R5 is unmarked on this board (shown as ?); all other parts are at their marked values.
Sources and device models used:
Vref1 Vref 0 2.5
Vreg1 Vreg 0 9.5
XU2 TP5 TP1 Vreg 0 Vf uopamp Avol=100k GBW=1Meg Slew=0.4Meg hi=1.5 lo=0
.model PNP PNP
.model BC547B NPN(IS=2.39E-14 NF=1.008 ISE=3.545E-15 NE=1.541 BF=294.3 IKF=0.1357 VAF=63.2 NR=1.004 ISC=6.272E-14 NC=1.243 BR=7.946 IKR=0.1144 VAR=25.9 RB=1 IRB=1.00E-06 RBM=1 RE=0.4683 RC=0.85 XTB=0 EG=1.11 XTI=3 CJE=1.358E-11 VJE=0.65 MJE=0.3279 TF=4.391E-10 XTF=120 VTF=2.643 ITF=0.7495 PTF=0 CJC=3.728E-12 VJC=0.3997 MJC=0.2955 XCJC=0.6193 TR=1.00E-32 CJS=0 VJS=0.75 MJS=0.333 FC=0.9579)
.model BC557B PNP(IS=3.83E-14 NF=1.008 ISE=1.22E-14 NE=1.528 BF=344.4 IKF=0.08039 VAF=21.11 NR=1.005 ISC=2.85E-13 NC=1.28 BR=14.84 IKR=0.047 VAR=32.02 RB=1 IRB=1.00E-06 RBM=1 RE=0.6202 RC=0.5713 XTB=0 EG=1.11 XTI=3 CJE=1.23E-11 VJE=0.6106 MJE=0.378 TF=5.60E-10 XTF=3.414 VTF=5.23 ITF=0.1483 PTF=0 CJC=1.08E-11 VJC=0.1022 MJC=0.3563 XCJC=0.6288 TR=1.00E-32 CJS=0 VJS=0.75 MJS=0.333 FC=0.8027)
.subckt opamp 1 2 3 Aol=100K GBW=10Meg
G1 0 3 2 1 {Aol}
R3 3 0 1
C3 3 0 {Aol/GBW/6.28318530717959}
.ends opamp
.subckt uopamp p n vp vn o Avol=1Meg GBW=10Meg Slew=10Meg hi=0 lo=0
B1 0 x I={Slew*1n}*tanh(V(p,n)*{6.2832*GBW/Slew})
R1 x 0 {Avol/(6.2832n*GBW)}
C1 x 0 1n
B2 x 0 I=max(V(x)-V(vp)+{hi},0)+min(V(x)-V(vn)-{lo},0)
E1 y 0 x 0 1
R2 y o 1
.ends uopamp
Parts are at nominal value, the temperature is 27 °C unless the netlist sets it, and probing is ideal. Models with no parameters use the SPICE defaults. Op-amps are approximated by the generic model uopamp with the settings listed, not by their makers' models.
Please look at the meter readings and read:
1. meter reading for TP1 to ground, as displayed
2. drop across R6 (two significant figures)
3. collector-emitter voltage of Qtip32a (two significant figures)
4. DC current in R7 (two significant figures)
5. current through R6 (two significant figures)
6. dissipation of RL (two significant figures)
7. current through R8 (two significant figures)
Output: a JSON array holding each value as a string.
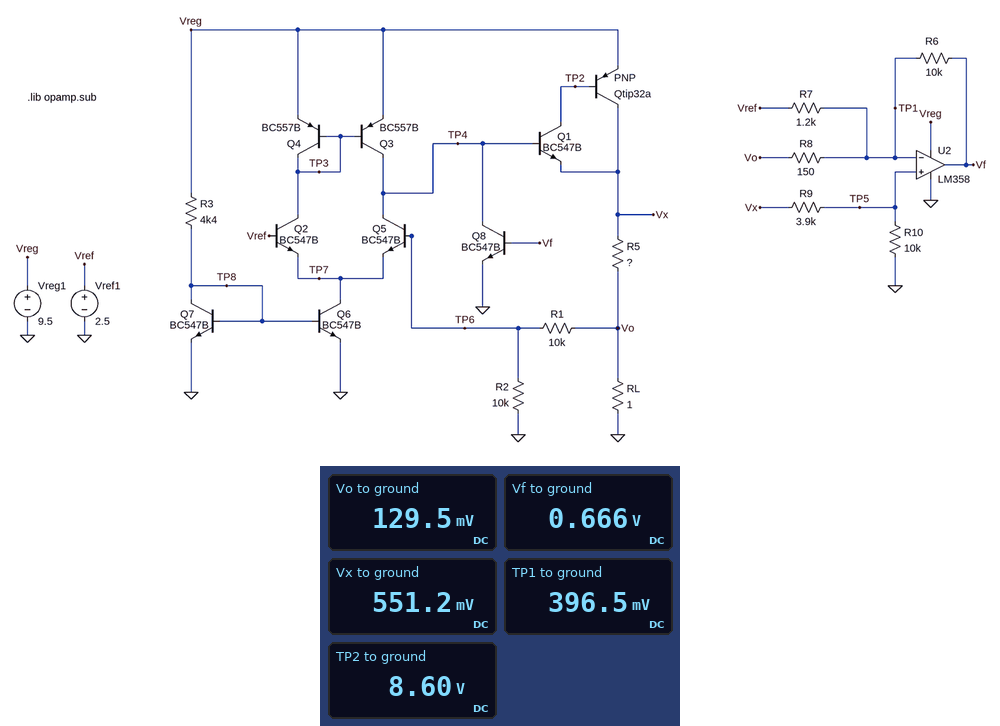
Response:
["396.5 mV", "270 mV", "-8.9 V", "1.8 mA", "27 µA", "17 mW", "1.8 mA"]
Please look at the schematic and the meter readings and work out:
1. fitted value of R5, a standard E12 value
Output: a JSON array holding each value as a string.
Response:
["3.3 Ω"]
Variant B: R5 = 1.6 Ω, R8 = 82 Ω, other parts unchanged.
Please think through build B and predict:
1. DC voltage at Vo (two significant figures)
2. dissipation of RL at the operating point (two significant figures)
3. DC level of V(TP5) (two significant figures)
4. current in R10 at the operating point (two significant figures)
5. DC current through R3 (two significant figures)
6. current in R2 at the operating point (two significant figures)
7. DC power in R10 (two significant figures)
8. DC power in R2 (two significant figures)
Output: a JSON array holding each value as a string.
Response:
["180 mV", "31 mW", "330 mV", "33 µA", "2.0 mA", "8.8 µA", "11 µW", "780 nW"]
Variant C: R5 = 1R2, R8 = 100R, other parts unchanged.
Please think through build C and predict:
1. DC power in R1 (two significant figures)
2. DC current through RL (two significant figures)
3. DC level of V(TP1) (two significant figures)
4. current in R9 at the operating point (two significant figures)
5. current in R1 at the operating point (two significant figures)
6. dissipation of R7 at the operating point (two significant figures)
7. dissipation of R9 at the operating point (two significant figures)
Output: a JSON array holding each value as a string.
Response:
["2.2 µW", "300 mA", "470 mV", "47 µA", "15 µA", "3.4 mW", "8.5 µW"]
